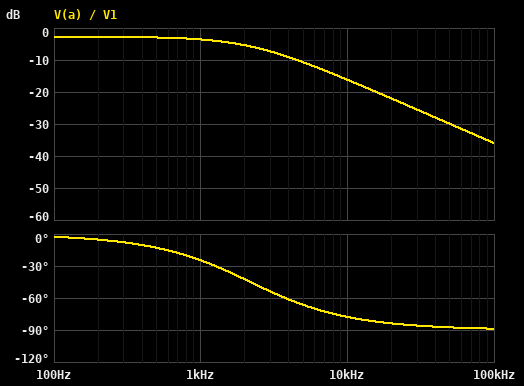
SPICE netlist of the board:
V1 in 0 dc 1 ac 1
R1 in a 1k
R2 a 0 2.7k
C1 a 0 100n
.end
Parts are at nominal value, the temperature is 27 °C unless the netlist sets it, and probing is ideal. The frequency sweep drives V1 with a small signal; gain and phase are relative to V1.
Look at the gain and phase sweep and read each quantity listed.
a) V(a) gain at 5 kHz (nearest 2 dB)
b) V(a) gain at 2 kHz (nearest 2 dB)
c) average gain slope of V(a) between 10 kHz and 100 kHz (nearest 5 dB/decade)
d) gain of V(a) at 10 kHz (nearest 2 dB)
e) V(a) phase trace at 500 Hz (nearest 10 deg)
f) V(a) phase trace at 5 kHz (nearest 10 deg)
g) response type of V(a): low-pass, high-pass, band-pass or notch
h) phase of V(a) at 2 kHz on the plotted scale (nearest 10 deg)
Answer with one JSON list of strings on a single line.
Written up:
["-10 dB", "-6 dB", "-20 dB/decade", "-16 dB", "-10 deg", "-70 deg", "low-pass", "-40 deg"]
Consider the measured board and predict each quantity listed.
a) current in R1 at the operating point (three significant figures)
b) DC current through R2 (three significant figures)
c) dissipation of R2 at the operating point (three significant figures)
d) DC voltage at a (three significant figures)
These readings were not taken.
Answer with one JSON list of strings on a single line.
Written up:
["270 µA", "270 µA", "197 µW", "730 mV"]
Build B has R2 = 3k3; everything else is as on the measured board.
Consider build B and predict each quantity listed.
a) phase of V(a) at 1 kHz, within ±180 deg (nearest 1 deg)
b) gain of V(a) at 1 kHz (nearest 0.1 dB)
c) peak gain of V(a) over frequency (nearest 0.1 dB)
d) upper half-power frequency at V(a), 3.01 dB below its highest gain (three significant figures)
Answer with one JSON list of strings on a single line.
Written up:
["-26 deg", "-3.2 dB", "-2.3 dB", "2.07 kHz"]
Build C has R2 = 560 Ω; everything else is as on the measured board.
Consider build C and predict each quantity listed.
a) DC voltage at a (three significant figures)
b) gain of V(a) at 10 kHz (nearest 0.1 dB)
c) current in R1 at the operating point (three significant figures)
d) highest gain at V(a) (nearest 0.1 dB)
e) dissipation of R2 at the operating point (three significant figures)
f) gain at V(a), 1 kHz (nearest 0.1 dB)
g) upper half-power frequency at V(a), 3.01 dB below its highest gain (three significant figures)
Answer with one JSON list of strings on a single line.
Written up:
["359 mV", "-16.7 dB", "641 µA", "-8.9 dB", "230 µW", "-9.1 dB", "4.43 kHz"]
